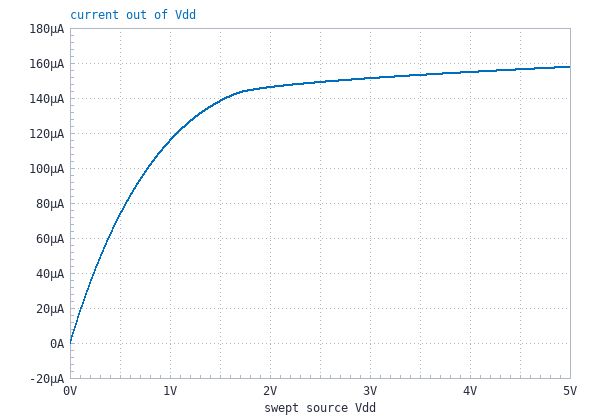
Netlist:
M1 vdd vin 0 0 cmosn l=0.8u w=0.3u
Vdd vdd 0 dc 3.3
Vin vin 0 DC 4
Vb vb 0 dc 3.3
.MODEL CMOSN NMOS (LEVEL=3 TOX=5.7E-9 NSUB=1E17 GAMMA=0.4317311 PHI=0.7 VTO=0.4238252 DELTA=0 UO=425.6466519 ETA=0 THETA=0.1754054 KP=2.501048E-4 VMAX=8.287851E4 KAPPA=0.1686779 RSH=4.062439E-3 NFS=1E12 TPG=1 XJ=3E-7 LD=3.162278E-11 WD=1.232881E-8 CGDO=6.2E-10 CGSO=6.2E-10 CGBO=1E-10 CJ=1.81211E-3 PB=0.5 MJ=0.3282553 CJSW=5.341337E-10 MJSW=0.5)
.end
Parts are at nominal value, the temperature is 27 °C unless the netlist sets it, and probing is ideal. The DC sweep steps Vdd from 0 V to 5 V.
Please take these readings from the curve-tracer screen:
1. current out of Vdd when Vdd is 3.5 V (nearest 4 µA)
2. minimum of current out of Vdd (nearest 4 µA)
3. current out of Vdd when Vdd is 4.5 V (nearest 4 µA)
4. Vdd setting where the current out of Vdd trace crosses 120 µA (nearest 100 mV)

152 µA
0 A
156 µA
1.1 V
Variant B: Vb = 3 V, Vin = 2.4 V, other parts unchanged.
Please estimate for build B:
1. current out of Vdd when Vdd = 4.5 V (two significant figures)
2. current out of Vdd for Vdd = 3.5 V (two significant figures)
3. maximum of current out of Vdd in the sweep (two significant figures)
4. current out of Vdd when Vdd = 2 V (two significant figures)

72 µA
71 µA
73 µA
68 µA
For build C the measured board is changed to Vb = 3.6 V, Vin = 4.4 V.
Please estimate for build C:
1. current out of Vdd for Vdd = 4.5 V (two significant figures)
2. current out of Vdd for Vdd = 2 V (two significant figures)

180 µA
170 µA
